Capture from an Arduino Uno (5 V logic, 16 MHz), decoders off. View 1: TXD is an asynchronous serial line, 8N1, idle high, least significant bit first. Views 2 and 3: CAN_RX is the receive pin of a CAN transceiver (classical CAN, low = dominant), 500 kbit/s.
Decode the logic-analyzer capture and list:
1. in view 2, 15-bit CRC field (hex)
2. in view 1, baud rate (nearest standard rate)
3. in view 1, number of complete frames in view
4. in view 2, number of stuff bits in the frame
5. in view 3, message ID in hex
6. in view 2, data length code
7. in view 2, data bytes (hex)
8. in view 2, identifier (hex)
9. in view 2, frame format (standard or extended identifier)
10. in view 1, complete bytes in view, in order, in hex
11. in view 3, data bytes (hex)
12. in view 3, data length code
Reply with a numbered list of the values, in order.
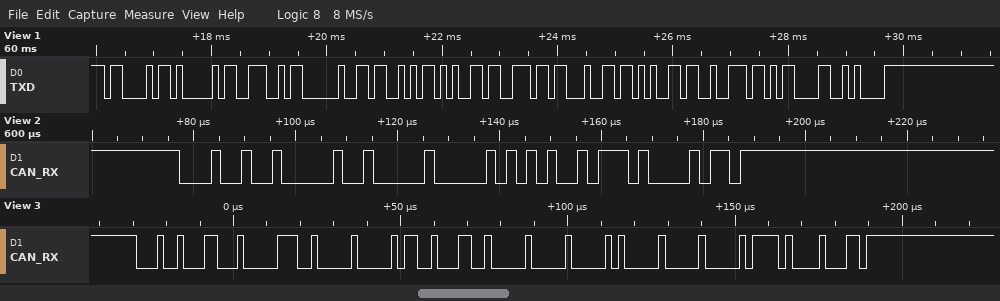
1. 0x2E85
2. 9600 baud
3. 12
4. 3
5. 0x123
6. 2
7. 00 2A
8. 0x124
9. standard
10. 43 41 4E 20 53 65 6E 64 65 72 0D 0A
11. 32 00 32 32 00 01 00 00
12. 8
